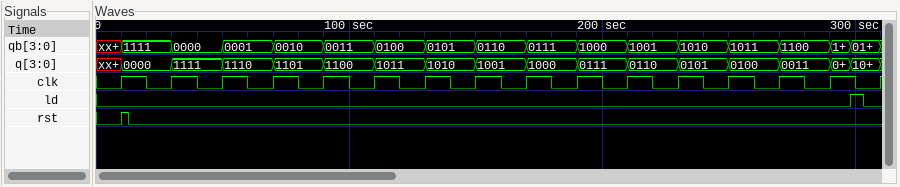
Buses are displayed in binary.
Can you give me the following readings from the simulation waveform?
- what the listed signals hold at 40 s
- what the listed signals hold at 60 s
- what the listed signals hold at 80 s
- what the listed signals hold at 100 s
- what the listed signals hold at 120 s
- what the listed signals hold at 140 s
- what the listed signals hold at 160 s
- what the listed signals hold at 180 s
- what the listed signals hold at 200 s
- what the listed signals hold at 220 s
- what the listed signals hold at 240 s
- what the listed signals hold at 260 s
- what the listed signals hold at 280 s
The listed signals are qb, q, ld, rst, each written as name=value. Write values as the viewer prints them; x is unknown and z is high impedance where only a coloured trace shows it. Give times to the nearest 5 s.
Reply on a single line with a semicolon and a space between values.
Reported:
qb=0000, q=1111, ld=0, rst=0; qb=0001, q=1110, ld=0, rst=0; qb=0010, q=1101, ld=0, rst=0; qb=0011, q=1100, ld=0, rst=0; qb=0100, q=1011, ld=0, rst=0; qb=0101, q=1010, ld=0, rst=0; qb=0110, q=1001, ld=0, rst=0; qb=0111, q=1000, ld=0, rst=0; qb=1000, q=0111, ld=0, rst=0; qb=1001, q=0110, ld=0, rst=0; qb=1010, q=0101, ld=0, rst=0; qb=1011, q=0100, ld=0, rst=0; qb=1100, q=0011, ld=0, rst=0
